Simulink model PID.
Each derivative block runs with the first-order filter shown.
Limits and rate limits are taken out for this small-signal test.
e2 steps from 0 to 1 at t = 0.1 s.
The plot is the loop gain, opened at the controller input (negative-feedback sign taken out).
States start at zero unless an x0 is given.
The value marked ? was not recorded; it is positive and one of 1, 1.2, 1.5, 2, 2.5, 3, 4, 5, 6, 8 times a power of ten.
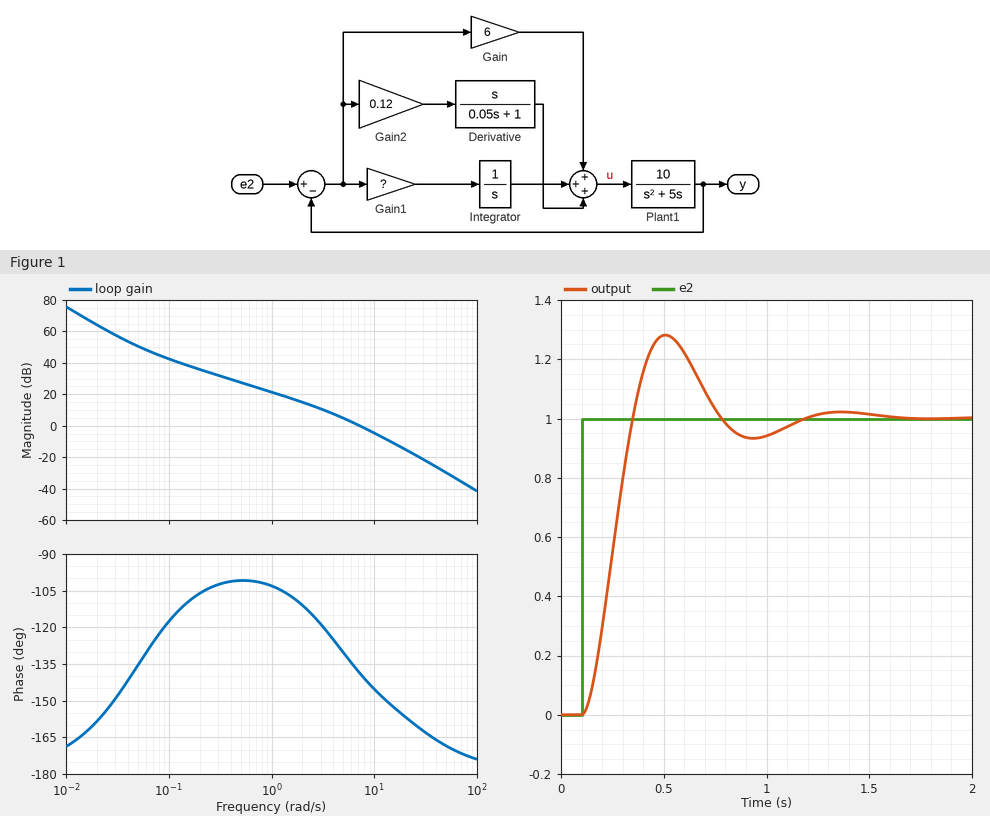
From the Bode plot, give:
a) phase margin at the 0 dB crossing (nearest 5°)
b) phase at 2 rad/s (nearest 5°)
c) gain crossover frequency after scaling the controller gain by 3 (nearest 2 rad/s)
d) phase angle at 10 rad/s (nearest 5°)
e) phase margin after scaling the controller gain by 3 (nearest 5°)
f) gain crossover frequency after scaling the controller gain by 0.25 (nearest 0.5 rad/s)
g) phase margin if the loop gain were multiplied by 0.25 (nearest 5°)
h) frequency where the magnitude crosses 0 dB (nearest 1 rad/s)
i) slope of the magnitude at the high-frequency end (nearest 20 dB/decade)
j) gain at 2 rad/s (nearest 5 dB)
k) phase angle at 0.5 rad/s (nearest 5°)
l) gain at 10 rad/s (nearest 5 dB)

40°
-110°
14 rad/s
-145°
30°
2.5 rad/s
65°
7 rad/s
-40 dB/decade
15 dB
-100°
-5 dB
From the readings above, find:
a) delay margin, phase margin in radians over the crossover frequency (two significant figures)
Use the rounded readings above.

0.100 s
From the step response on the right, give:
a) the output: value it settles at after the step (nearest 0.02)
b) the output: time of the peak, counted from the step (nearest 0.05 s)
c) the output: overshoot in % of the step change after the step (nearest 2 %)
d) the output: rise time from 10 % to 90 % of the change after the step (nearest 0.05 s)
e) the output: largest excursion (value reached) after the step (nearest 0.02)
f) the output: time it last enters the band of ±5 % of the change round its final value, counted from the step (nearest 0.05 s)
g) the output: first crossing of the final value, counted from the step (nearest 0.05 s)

1.00
0.40 s
28 %
0.15 s
1.28
0.95 s
0.25 s
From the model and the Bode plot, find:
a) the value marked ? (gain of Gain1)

0.3
